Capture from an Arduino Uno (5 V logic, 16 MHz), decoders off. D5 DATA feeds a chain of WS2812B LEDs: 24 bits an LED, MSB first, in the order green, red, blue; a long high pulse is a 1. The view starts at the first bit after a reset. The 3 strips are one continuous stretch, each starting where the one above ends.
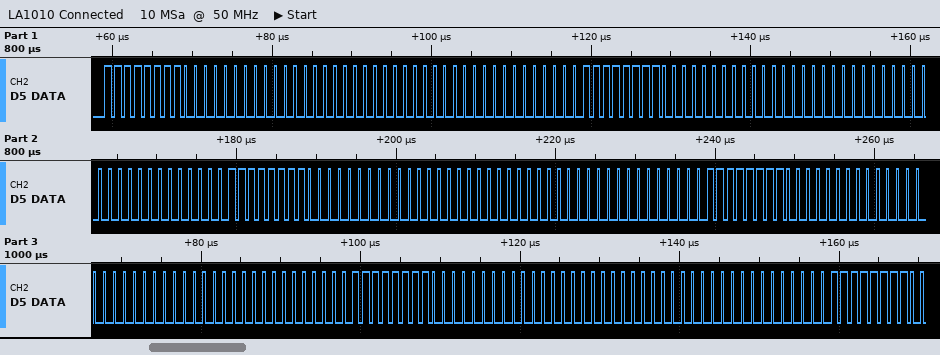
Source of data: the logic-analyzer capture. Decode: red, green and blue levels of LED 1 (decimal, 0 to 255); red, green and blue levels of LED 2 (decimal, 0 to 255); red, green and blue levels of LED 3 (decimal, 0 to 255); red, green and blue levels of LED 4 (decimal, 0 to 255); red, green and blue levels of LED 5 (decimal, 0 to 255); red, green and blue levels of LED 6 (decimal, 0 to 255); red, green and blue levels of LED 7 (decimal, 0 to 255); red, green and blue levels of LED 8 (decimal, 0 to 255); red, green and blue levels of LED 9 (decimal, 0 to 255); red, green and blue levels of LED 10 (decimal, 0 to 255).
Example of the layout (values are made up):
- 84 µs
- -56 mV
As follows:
- 0, 255, 0
- 0, 0, 0
- 0, 255, 0
- 0, 0, 0
- 0, 255, 0
- 0, 0, 0
- 0, 255, 0
- 0, 0, 0
- 0, 255, 0
- 0, 0, 0
